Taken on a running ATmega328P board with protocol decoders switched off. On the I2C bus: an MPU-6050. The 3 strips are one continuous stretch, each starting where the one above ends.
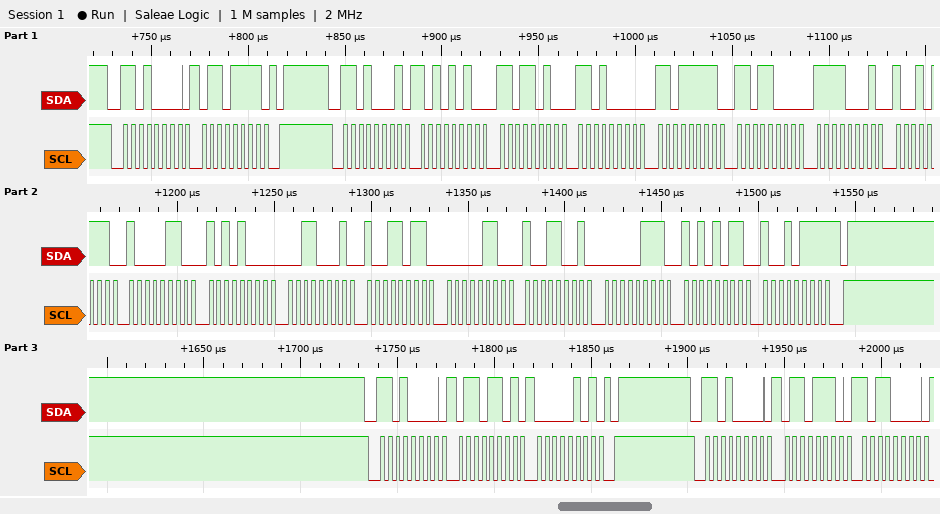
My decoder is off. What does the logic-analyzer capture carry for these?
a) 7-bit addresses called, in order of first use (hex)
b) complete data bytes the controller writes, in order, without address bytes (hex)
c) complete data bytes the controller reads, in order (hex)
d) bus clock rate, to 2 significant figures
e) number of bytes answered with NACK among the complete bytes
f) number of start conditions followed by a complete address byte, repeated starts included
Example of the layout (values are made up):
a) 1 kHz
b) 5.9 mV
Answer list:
a) 0x68
b) 6F 6D 05 6E B0
c) AA DA D0 DF D8 F1 97 86 A8 31 9B 06 99 07 AB 97
d) 250 kHz
e) 1
f) 4
